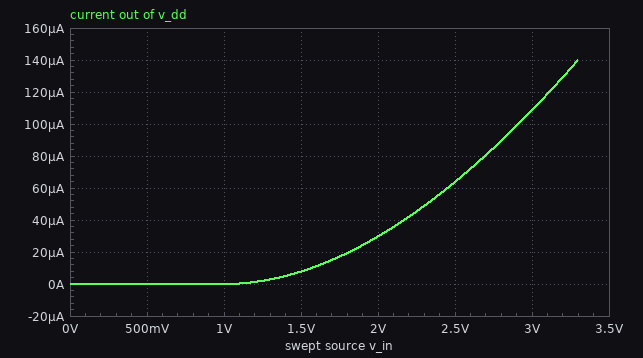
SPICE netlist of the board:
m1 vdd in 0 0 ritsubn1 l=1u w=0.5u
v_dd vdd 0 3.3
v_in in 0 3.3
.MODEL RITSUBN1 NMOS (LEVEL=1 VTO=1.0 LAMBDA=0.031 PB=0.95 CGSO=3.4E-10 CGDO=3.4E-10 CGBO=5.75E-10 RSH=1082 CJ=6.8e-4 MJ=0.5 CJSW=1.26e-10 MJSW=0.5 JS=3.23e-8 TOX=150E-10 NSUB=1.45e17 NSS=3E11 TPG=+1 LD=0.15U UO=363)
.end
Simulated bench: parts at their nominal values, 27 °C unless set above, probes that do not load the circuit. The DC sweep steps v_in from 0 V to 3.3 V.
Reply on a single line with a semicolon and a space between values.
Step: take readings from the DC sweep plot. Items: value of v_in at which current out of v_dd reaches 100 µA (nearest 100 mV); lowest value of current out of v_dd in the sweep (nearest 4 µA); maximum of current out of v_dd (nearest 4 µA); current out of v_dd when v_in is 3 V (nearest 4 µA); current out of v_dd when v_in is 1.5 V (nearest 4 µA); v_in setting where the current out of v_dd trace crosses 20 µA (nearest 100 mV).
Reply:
2.9 V; 0 A; 140 µA; 108 µA; 8 µA; 1.8 V
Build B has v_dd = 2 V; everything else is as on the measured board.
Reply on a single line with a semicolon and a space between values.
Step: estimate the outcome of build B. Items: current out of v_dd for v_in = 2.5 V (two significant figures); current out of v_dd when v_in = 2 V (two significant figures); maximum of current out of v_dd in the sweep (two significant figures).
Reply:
62 µA; 29 µA; 130 µA
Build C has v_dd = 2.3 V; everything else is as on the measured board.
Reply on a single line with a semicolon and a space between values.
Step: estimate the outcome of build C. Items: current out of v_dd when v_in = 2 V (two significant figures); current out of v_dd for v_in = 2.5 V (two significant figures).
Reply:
29 µA; 62 µA
